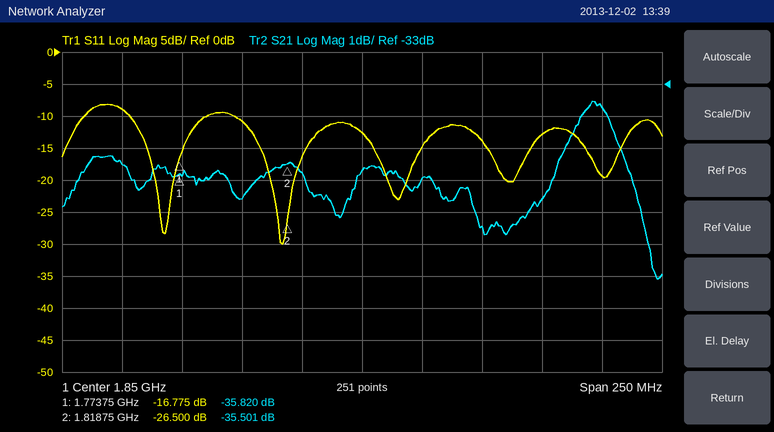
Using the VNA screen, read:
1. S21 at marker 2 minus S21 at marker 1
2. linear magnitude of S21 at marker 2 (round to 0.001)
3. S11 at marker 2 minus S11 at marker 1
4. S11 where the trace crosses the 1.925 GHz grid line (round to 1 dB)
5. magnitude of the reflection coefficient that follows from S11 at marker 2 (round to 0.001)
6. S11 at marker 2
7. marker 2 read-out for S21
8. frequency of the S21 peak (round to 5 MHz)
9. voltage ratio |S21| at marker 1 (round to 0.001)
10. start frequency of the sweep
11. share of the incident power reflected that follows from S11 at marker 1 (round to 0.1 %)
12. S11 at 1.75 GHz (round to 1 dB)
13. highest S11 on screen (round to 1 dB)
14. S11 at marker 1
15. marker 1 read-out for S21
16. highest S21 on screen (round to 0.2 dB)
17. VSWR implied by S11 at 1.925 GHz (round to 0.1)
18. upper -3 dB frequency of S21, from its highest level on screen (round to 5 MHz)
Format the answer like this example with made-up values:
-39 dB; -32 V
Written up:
0.319 dB; 0.017; -9.725 dB; -13 dB; 0.047; -26.500 dB; -35.501 dB; 1.945 GHz; 0.016; 1.725 GHz; 2.1 %; -9 dB; -8 dB; -16.775 dB; -35.820 dB; -33.6 dB; 1.6; 1.965 GHz
